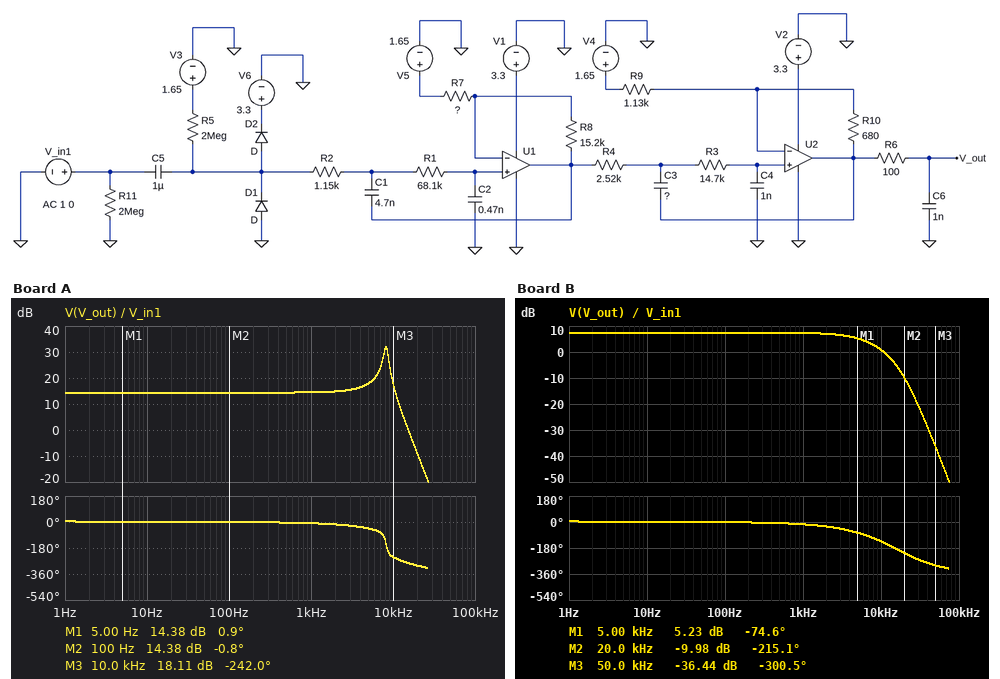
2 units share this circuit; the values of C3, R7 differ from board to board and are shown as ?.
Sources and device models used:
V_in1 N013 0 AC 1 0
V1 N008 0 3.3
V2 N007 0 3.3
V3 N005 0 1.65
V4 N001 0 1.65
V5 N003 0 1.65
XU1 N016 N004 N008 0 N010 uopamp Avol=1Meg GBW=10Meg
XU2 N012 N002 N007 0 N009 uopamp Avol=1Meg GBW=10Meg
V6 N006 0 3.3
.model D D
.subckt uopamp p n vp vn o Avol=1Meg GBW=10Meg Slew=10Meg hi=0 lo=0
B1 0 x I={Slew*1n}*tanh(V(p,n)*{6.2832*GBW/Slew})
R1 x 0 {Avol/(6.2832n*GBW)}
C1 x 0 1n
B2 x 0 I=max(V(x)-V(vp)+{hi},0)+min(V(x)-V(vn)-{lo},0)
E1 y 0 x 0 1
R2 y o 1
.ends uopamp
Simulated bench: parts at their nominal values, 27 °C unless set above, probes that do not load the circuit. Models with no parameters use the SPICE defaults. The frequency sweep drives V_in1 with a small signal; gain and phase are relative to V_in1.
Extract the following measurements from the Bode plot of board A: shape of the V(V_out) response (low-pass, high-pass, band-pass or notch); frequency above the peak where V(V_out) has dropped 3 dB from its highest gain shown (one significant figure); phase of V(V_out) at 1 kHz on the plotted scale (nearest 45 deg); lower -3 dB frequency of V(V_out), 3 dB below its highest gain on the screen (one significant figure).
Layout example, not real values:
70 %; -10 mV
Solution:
band-pass; 9 kHz; 0 deg; 8 kHz
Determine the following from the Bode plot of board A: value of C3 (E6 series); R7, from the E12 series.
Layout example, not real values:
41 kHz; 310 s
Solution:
10 nF; 6.8 kΩ
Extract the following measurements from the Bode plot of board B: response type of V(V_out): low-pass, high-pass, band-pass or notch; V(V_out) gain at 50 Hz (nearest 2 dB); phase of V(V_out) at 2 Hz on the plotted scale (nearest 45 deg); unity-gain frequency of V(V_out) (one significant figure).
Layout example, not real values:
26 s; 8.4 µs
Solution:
low-pass; 8 dB; 0 deg; 10 kHz
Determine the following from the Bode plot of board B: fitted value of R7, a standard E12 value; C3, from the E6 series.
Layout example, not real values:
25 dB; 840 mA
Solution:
33 kΩ; 2.2 nF
